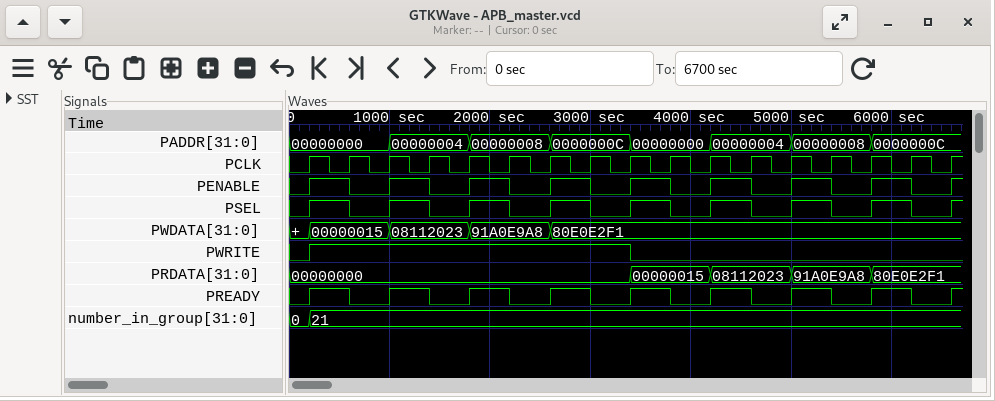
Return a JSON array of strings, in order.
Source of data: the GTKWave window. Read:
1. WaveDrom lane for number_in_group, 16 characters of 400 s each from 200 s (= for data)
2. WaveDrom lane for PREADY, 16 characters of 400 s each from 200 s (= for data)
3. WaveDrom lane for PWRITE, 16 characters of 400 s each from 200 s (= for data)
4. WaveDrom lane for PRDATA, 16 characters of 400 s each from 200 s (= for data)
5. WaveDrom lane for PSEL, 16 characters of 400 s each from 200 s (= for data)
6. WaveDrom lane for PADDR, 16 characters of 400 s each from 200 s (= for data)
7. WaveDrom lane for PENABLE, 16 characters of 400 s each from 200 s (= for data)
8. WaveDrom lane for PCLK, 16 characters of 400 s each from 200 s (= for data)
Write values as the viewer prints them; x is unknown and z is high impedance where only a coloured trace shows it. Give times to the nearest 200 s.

["{name: 'number_in_group', wave: '=...............', data: '21'}", "{name: 'PREADY', wave: '1010101010101010'}", "{name: 'PWRITE', wave: '1.......0.......'}", "{name: 'PRDATA', wave: '=.......=.=.=.=.', data: '00000000 00000015 08112023 91A0E9A8 80E0E2F1'}", "{name: 'PSEL', wave: '1010101010101010'}", "{name: 'PADDR', wave: '=.=.=.=.=.=.=.=.', data: '00000000 00000004 00000008 0000000C 00000000 00000004 00000008 0000000C'}", "{name: 'PENABLE', wave: '1010101010101010'}", "{name: 'PCLK', wave: 'p...............'}"]
